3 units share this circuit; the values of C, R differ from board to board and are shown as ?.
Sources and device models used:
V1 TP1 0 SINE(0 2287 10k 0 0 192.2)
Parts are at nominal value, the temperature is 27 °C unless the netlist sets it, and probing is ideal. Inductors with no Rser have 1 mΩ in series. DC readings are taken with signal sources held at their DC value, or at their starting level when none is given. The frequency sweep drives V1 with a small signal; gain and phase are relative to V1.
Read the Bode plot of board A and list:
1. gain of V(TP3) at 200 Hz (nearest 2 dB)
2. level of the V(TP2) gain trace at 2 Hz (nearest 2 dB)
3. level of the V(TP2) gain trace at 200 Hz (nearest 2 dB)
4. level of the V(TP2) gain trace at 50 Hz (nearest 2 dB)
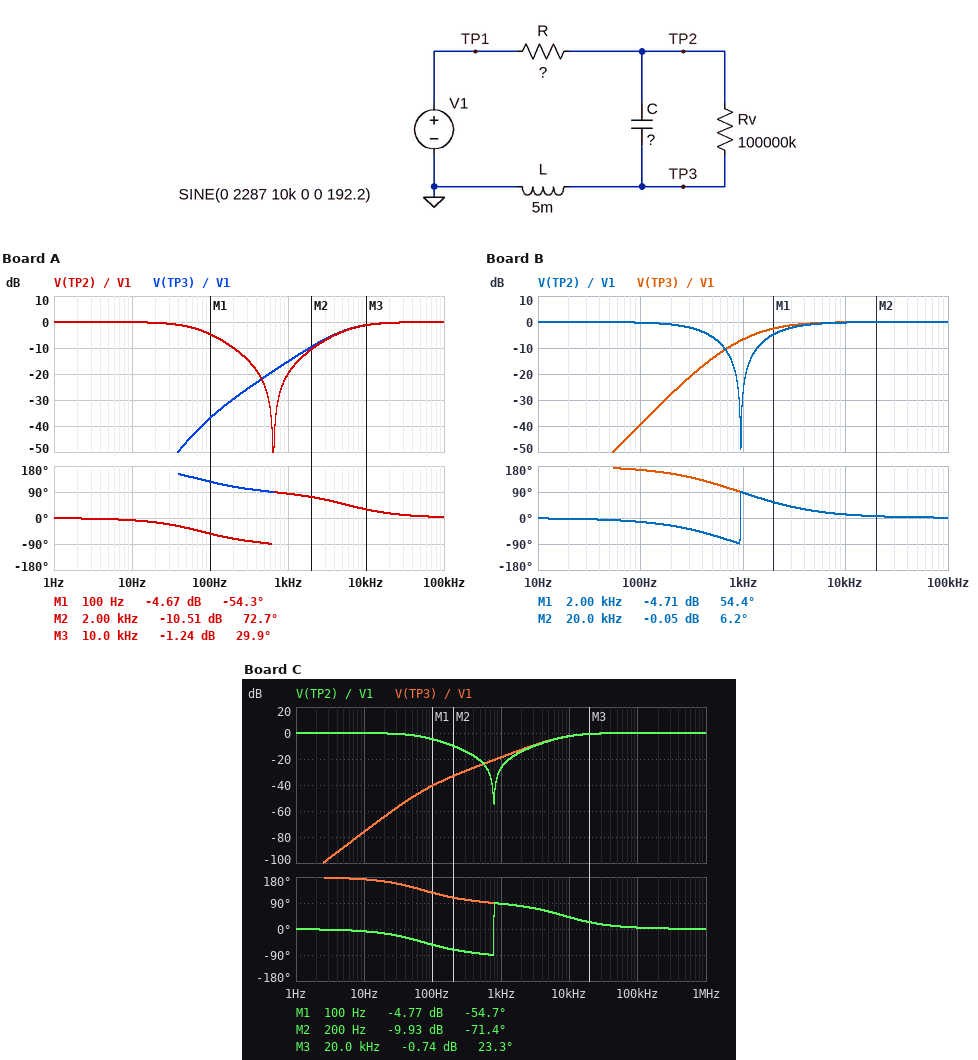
-30 dB
0 dB
-10 dB
-2 dB
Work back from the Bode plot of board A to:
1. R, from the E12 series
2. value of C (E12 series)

180 Ω
12 µF
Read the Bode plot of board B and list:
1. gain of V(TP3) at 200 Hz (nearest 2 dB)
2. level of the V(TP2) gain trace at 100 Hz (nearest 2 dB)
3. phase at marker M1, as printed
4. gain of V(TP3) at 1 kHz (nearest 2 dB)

-28 dB
0 dB
54.4 deg
-6 dB
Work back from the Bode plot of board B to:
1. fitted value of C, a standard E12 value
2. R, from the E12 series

5.6 µF
68 Ω
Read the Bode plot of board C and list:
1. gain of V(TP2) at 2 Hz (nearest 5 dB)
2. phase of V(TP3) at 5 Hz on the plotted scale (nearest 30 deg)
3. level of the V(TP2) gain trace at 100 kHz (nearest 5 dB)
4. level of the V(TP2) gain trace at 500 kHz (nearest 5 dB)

0 dB
180 deg
0 dB
0 dB
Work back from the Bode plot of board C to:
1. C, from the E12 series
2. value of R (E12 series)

8.2 µF
270 Ω
